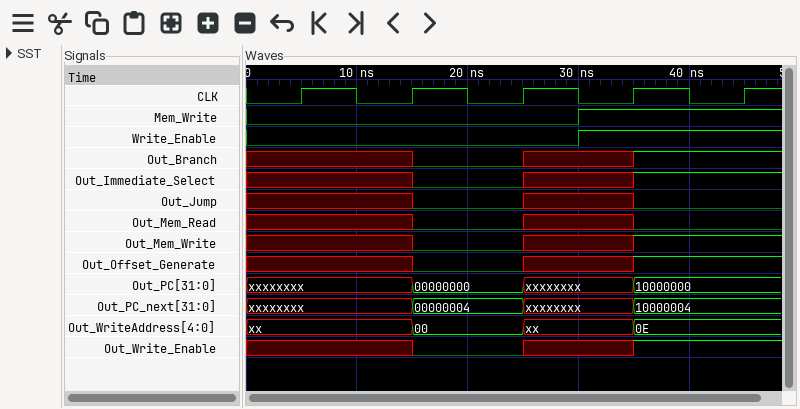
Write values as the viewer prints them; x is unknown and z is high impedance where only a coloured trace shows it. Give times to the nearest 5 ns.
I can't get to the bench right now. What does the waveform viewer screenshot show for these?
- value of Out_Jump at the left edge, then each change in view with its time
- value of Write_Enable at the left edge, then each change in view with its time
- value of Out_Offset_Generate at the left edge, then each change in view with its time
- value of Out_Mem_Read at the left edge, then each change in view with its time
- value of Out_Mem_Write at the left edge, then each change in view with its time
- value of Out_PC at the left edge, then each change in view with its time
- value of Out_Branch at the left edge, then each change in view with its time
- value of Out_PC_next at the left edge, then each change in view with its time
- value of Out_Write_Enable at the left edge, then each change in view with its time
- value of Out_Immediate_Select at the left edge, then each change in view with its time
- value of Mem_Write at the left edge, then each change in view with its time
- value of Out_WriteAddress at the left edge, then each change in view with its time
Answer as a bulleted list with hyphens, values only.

- x, 0 at 15 ns, x at 25 ns, 0 at 35 ns
- 0, 1 at 30 ns
- x, 0 at 15 ns, x at 25 ns, 1 at 35 ns
- x, 0 at 15 ns, x at 25 ns, 0 at 35 ns
- x, 0 at 15 ns, x at 25 ns, 1 at 35 ns
- xxxxxxxx, 00000000 at 15 ns, xxxxxxxx at 25 ns, 10000000 at 35 ns
- x, 0 at 15 ns, x at 25 ns, 1 at 35 ns
- xxxxxxxx, 00000004 at 15 ns, xxxxxxxx at 25 ns, 10000004 at 35 ns
- x, 0 at 15 ns, x at 25 ns, 1 at 35 ns
- x, 0 at 15 ns, x at 25 ns, 1 at 35 ns
- 0, 1 at 30 ns
- xx, 00 at 15 ns, xx at 25 ns, 0E at 35 ns
